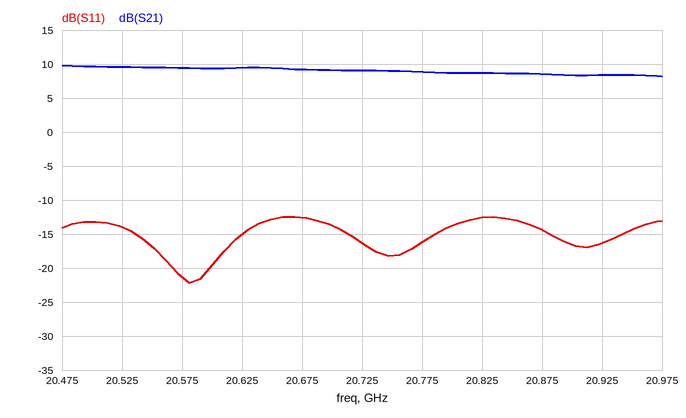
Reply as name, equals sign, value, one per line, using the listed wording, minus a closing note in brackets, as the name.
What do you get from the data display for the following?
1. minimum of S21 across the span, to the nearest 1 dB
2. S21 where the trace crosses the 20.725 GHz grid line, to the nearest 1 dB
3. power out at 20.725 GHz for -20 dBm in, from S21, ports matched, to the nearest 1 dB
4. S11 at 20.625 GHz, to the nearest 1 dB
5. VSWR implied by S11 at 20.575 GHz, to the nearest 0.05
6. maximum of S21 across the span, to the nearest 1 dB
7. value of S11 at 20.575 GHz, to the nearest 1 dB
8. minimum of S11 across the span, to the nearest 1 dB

minimum of S21 across the span, to the nearest 1 dB = 8 dB
S21 where the trace crosses the 20.725 GHz grid line, to the nearest 1 dB = 9 dB
power out at 20.725 GHz for -20 dBm in, from S21, ports matched, to the nearest 1 dB = -11 dBm
S11 at 20.625 GHz, to the nearest 1 dB = -15 dB
VSWR implied by S11 at 20.575 GHz, to the nearest 0.05 = 1.20
maximum of S21 across the span, to the nearest 1 dB = 10 dB
value of S11 at 20.575 GHz, to the nearest 1 dB = -21 dB
minimum of S11 across the span, to the nearest 1 dB = -22 dB
